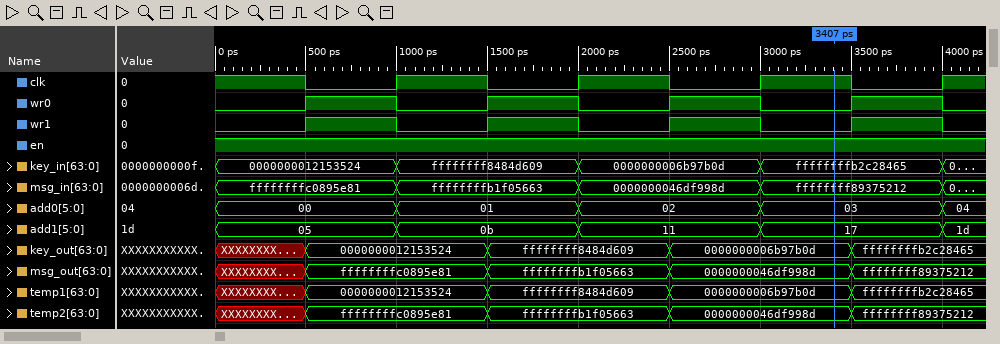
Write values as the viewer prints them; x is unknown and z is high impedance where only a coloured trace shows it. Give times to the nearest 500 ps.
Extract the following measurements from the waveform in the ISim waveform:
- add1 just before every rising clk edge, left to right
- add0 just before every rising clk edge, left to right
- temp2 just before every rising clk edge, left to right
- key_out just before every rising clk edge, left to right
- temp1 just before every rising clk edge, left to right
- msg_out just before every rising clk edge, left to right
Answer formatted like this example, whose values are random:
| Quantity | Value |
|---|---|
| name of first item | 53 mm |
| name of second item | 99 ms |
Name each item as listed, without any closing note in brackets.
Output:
| Quantity | Value |
|---|---|
| add1 just before every rising clk edge, left to right | 05, 0b, 11, 17 |
| add0 just before every rising clk edge, left to right | 00, 01, 02, 03 |
| temp2 just before every rising clk edge, left to right | ffffffffc0895e81, ffffffffb1f05663, 0000000046df998d, ffffffff89375212 |
| key_out just before every rising clk edge, left to right | 0000000012153524, ffffffff8484d609, 0000000006b97b0d, ffffffffb2c28465 |
| temp1 just before every rising clk edge, left to right | 0000000012153524, ffffffff8484d609, 0000000006b97b0d, ffffffffb2c28465 |
| msg_out just before every rising clk edge, left to right | ffffffffc0895e81, ffffffffb1f05663, 0000000046df998d, ffffffff89375212 |
